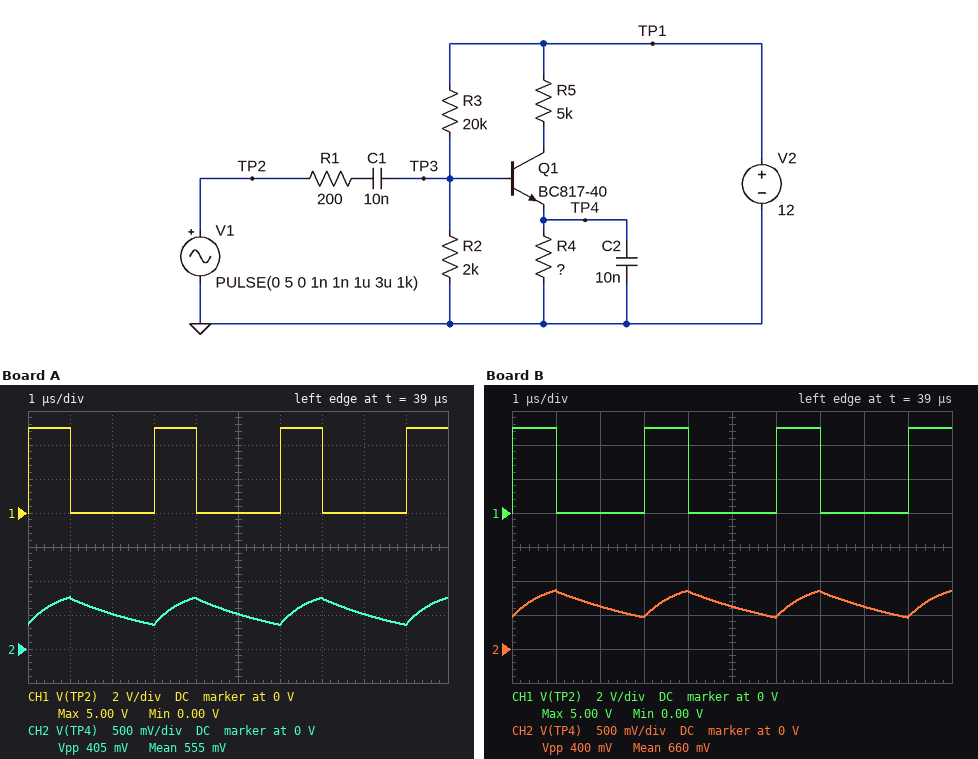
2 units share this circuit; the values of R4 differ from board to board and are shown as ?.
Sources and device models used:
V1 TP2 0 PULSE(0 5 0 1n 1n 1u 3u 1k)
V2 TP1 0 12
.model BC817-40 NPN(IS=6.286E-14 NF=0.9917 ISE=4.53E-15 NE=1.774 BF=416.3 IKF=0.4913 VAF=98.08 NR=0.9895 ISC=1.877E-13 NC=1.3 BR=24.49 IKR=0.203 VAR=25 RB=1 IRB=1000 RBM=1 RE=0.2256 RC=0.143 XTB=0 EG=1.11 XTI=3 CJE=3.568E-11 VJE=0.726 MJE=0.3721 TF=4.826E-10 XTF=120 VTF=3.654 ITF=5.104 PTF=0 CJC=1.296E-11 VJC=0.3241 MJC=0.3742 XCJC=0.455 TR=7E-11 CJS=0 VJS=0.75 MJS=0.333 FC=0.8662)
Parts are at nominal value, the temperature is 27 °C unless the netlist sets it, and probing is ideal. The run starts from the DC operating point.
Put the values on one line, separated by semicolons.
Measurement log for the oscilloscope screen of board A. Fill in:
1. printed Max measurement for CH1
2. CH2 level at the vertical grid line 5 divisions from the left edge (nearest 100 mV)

5.00 V; 500 mV
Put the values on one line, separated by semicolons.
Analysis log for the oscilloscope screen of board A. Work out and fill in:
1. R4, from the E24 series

270 Ω
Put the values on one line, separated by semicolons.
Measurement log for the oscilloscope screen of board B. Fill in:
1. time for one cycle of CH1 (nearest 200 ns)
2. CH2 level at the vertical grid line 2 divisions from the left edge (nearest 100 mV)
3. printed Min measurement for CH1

3.0 µs; 600 mV; 0.00 V
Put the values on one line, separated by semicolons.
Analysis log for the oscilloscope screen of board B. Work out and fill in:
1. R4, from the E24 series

330 Ω
